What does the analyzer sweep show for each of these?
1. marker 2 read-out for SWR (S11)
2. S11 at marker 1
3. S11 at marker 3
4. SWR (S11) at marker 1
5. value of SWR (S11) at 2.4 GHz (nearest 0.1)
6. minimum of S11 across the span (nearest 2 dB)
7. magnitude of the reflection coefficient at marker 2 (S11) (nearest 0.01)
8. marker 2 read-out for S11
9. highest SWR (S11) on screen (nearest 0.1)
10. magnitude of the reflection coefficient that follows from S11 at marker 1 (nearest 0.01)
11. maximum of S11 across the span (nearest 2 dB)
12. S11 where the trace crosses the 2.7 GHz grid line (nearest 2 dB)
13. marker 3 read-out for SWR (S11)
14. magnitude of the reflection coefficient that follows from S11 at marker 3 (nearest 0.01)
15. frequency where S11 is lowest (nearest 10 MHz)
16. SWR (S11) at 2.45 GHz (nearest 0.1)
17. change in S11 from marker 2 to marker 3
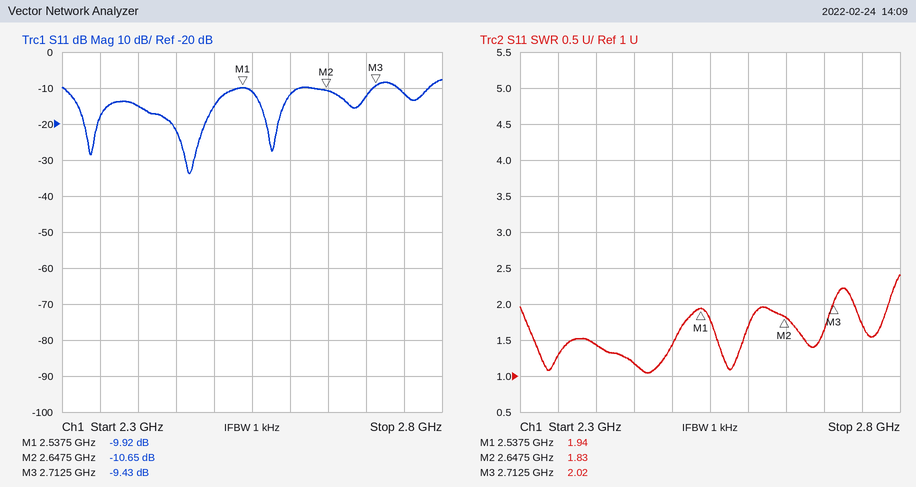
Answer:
1.83
-9.92 dB
-9.43 dB
1.94
1.4
-34 dB
0.29
-10.65 dB
2.4
0.32
-8 dB
-12 dB
2.02
0.34
2.47 GHz
1.2
1.22 dB
